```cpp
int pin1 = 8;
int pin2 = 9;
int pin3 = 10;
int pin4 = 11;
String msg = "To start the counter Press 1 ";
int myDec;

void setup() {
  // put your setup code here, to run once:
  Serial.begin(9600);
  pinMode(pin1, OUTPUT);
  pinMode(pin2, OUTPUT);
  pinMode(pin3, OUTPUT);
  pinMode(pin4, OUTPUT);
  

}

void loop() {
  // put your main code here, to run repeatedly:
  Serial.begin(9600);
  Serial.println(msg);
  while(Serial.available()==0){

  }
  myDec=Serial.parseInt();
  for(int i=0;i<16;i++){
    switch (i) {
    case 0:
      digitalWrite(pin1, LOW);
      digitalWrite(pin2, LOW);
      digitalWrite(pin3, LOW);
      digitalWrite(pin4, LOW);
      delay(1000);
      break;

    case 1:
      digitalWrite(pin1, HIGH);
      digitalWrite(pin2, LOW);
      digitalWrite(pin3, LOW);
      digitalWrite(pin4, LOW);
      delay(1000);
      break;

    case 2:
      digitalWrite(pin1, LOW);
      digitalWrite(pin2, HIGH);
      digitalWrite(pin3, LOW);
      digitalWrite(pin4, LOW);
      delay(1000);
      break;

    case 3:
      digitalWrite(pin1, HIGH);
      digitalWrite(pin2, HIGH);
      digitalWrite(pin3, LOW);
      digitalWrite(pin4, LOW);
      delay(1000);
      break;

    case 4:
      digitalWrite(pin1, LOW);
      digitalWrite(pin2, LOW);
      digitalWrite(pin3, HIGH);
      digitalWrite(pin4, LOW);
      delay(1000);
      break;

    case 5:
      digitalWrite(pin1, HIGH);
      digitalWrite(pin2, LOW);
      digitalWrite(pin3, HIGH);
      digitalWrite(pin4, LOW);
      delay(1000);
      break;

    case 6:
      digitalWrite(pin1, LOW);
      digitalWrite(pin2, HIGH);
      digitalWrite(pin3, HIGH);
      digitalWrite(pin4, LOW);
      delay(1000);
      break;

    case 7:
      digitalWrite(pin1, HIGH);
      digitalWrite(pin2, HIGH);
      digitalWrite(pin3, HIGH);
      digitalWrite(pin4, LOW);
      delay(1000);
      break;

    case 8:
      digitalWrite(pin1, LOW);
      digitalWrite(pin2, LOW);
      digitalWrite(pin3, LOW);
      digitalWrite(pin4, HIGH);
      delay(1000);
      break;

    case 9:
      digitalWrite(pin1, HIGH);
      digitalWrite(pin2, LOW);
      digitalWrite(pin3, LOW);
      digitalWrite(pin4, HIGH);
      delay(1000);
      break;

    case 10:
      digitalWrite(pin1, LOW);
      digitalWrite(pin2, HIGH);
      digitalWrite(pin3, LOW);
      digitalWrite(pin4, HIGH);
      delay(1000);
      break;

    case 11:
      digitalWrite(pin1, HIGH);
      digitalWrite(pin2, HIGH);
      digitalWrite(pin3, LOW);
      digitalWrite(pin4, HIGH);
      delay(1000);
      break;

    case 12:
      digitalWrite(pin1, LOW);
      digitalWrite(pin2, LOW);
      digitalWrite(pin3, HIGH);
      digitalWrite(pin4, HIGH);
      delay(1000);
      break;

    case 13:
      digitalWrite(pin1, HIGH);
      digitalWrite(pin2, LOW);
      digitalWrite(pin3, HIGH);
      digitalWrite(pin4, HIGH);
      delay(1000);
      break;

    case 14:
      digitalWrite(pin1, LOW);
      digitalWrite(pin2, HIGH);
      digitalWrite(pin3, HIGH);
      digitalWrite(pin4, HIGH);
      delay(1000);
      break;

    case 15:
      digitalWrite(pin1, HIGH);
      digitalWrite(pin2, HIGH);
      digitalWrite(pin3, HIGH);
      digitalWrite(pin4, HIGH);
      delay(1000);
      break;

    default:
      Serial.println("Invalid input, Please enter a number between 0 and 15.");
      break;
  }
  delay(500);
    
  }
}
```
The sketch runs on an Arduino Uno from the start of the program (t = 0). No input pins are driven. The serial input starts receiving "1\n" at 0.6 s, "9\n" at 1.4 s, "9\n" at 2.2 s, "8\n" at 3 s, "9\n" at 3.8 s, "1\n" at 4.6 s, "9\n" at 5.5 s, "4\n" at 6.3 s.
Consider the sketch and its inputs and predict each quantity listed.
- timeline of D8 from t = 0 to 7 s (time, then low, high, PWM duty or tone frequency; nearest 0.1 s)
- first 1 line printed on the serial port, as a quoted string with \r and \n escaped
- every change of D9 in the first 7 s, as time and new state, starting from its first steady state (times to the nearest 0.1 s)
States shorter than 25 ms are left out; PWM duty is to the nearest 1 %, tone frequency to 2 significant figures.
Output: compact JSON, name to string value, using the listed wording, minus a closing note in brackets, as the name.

{"timeline of D8 from t = 0 to 7 s": "0 s low; 2.1 s high; 3.6 s low; 5.1 s high; 6.6 s low", "first 1 line printed on the serial port, as a quoted string with \\r and \\n escaped": "\"To start the counter Press 1 \\r\\n\"", "every change of D9 in the first 7 s, as time and new state, starting from its first steady state": "0 s low; 3.6 s high; 6.6 s low"}
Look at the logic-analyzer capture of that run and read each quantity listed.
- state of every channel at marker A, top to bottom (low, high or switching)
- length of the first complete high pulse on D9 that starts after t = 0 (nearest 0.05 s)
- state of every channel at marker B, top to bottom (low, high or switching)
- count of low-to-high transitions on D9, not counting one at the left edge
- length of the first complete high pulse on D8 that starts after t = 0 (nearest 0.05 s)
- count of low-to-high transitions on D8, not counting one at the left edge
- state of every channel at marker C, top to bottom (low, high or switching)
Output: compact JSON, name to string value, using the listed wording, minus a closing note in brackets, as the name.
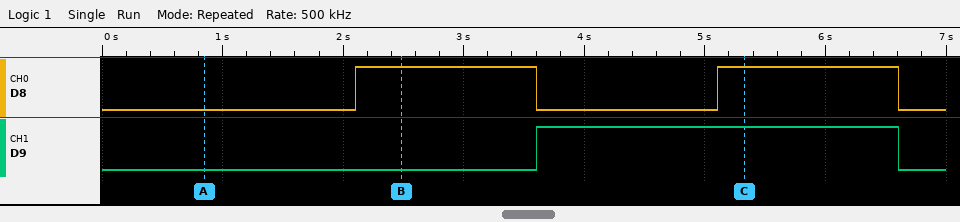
{"state of every channel at marker A, top to bottom": "D8 low, D9 low", "length of the first complete high pulse on D9 that starts after t = 0": "3.00 s", "state of every channel at marker B, top to bottom": "D8 high, D9 low", "count of low-to-high transitions on D9, not counting one at the left edge": "1", "length of the first complete high pulse on D8 that starts after t = 0": "1.50 s", "count of low-to-high transitions on D8, not counting one at the left edge": "2", "state of every channel at marker C, top to bottom": "D8 high, D9 high"}
